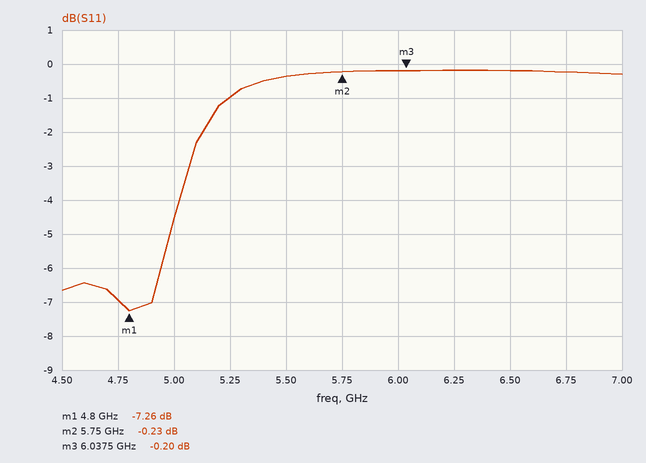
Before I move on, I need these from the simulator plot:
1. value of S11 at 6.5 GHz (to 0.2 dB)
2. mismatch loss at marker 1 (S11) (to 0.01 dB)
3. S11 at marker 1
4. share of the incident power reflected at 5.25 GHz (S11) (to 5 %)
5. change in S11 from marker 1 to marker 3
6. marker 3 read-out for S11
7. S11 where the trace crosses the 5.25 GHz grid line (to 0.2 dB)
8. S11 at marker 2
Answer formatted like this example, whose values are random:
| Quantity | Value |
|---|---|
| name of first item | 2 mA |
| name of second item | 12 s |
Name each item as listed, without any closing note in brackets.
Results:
| Quantity | Value |
|---|---|
| value of S11 at 6.5 GHz | -0.2 dB |
| mismatch loss at marker 1 (S11) | 0.90 dB |
| S11 at marker 1 | -7.26 dB |
| share of the incident power reflected at 5.25 GHz (S11) | 80 % |
| change in S11 from marker 1 to marker 3 | 7.06 dB |
| marker 3 read-out for S11 | -0.20 dB |
| S11 where the trace crosses the 5.25 GHz grid line | -1.0 dB |
| S11 at marker 2 | -0.23 dB |
